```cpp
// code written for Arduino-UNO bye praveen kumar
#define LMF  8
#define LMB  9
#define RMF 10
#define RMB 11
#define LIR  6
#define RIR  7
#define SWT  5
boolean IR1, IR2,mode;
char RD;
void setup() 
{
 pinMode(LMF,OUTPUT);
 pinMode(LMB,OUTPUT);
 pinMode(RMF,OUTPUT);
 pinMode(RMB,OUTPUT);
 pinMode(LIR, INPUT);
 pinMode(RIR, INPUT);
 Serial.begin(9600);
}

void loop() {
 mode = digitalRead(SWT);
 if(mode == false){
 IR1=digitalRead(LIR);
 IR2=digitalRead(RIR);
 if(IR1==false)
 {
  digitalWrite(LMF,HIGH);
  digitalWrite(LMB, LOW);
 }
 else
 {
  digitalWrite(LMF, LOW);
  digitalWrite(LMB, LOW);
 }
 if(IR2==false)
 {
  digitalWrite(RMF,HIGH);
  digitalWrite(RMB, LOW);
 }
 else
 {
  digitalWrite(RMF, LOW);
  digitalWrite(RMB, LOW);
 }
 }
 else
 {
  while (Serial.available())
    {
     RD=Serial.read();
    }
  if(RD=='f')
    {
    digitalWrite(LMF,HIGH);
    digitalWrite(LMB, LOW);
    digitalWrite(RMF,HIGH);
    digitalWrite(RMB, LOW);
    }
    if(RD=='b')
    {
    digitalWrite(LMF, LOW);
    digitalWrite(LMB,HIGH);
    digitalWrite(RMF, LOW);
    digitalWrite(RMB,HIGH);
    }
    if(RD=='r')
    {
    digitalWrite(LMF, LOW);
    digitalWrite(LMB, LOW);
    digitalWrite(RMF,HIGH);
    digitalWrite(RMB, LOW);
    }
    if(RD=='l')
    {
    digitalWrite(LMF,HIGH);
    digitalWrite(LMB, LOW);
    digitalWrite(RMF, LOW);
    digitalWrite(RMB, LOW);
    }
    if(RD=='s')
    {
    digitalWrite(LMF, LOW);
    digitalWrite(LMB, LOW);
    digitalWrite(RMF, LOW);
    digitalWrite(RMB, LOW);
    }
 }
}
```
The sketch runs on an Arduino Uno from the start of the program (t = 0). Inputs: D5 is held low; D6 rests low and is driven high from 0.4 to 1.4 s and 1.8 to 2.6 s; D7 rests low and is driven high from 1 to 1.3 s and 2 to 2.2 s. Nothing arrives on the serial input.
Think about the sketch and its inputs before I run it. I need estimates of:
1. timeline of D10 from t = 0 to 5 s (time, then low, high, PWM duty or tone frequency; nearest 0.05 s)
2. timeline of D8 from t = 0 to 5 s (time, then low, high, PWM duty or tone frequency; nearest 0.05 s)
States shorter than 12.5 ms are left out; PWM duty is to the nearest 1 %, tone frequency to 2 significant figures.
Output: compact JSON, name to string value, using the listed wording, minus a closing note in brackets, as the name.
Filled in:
{"timeline of D10 from t = 0 to 5 s": "0 s high; 1 s low; 1.3 s high; 2 s low; 2.2 s high", "timeline of D8 from t = 0 to 5 s": "0 s high; 0.4 s low; 1.4 s high; 1.8 s low; 2.6 s high"}
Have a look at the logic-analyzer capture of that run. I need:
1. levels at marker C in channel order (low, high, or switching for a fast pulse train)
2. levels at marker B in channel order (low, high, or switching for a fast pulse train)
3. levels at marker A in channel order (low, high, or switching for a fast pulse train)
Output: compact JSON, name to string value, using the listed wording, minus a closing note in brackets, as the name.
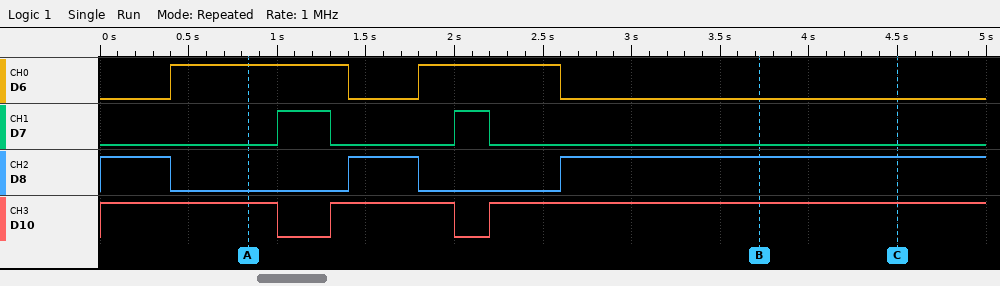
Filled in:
{"levels at marker C in channel order": "D6 low, D7 low, D8 high, D10 high", "levels at marker B in channel order": "D6 low, D7 low, D8 high, D10 high", "levels at marker A in channel order": "D6 high, D7 low, D8 low, D10 high"}
